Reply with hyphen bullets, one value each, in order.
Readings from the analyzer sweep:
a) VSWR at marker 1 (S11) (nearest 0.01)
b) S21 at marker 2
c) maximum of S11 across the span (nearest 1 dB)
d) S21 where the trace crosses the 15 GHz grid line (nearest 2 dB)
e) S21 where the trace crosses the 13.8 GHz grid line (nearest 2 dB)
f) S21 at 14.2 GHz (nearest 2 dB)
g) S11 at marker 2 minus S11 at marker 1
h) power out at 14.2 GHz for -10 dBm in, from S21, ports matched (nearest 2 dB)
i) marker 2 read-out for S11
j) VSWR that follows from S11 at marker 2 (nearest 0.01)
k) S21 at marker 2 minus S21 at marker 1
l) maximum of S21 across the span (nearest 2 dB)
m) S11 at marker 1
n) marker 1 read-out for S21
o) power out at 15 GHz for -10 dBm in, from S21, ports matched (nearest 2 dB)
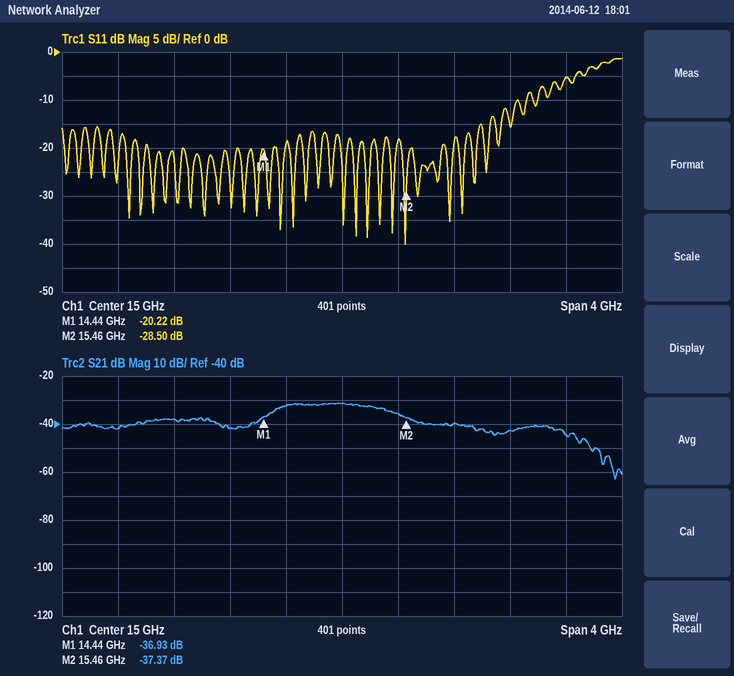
- 1.22
- -37.37 dB
- -1 dB
- -32 dB
- -38 dB
- -42 dB
- -8.28 dB
- -52 dBm
- -28.50 dB
- 1.08
- -0.44 dB
- -32 dB
- -20.22 dB
- -36.93 dB
- -42 dBm
